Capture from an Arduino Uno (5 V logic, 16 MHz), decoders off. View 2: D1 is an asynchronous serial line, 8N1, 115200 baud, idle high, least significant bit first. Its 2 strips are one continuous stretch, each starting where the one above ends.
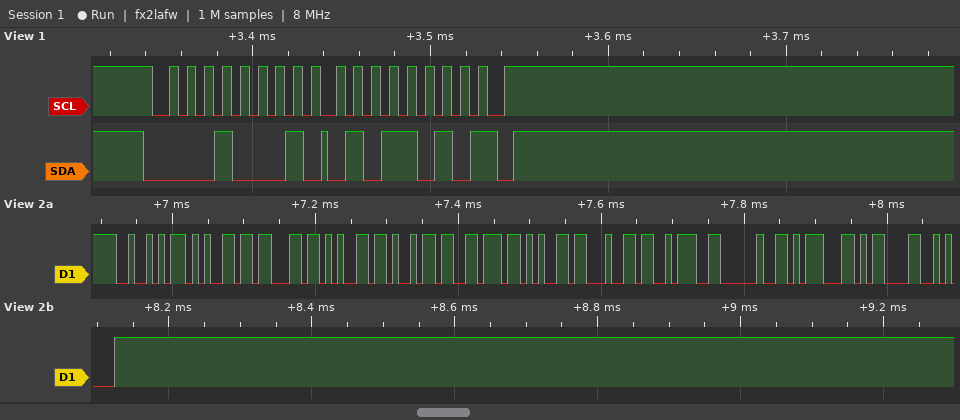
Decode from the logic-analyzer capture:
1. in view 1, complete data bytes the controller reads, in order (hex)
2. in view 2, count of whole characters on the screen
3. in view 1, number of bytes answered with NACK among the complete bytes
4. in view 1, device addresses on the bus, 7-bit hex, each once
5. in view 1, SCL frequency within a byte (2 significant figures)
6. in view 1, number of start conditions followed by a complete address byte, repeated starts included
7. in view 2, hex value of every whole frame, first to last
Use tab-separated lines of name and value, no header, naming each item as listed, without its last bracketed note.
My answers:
in view 1, complete data bytes the controller reads, in order	5A
in view 2, count of whole characters on the screen	13
in view 1, number of bytes answered with NACK among the complete bytes	1
in view 1, device addresses on the bus, 7-bit hex, each once	0x08
in view 1, SCL frequency within a byte	100 kHz
in view 1, number of start conditions followed by a complete address byte, repeated starts included	1
in view 2, hex value of every whole frame, first to last	52 65 63 65 69 76 65 64 3A 20 1D 0D 0A
